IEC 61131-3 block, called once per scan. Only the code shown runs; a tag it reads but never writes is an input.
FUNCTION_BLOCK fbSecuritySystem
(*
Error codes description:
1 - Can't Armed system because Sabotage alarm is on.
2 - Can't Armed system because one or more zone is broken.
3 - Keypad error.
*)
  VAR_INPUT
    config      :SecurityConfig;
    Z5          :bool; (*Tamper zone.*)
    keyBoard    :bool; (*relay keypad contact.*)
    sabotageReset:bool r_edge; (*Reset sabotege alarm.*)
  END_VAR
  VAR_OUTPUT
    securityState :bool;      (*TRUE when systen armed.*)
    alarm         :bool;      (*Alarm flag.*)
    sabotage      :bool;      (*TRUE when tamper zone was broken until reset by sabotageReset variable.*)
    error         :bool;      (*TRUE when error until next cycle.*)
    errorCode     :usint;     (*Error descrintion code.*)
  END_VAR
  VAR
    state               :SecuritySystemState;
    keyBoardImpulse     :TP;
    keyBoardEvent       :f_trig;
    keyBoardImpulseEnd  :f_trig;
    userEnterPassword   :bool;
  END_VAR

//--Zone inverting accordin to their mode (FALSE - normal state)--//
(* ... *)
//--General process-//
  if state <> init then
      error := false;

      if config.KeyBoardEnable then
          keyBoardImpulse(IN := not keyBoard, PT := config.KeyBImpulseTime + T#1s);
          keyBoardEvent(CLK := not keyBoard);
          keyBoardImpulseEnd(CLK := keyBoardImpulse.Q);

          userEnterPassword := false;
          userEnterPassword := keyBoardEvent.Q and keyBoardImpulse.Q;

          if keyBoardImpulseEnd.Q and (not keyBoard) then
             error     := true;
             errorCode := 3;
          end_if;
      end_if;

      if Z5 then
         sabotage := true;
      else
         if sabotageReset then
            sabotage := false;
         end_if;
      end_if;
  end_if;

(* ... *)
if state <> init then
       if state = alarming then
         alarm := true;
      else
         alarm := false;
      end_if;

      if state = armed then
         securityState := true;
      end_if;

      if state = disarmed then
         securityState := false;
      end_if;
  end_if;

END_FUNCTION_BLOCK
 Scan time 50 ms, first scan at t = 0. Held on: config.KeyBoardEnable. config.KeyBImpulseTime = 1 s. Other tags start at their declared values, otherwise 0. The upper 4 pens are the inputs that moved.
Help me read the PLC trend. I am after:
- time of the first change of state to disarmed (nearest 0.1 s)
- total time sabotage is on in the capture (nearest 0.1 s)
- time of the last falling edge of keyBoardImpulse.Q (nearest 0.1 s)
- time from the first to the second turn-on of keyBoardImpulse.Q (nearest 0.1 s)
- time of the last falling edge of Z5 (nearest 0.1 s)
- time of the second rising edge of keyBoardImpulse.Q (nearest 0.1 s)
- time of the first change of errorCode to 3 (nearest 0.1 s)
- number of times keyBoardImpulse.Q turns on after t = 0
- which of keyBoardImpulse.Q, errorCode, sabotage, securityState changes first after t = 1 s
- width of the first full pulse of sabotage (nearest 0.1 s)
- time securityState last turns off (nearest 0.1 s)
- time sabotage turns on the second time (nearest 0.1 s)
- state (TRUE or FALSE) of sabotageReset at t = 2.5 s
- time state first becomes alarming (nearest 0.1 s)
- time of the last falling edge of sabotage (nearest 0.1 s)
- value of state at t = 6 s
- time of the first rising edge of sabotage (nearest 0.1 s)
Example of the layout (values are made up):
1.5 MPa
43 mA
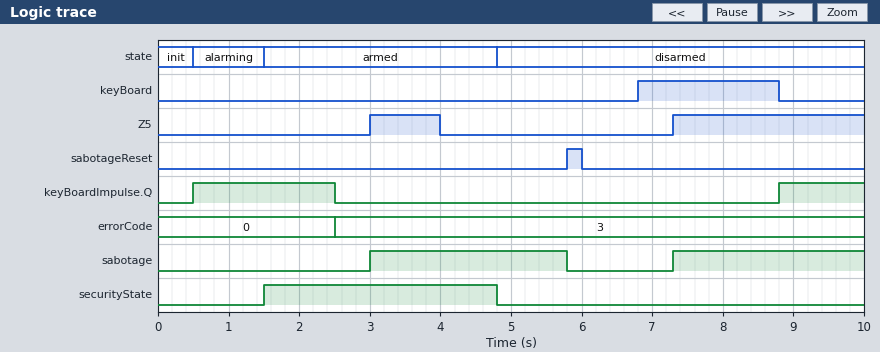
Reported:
4.8 s
5.5 s
2.5 s
8.3 s
4.0 s
8.8 s
2.5 s
2
securityState
2.8 s
4.8 s
7.3 s
FALSE
0.5 s
5.8 s
disarmed
3.0 s
